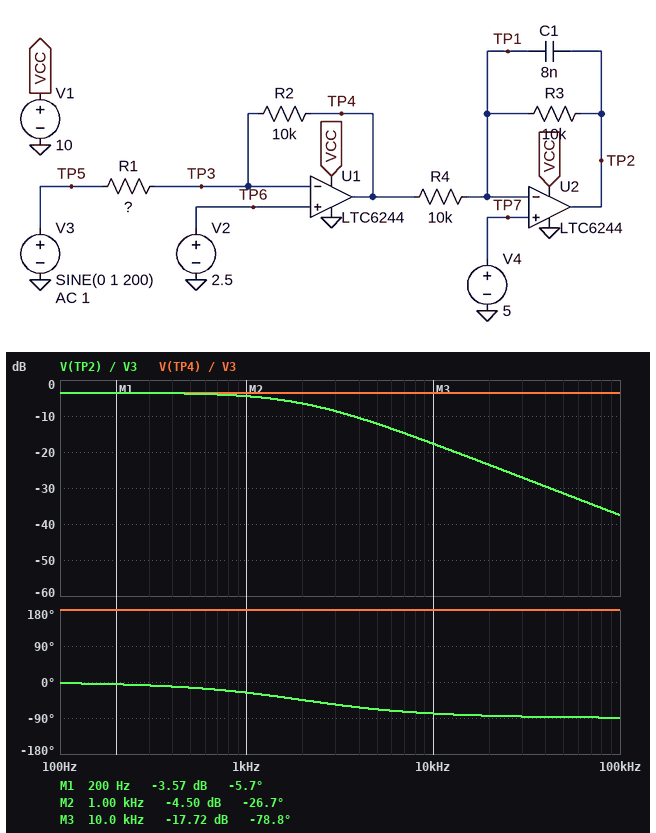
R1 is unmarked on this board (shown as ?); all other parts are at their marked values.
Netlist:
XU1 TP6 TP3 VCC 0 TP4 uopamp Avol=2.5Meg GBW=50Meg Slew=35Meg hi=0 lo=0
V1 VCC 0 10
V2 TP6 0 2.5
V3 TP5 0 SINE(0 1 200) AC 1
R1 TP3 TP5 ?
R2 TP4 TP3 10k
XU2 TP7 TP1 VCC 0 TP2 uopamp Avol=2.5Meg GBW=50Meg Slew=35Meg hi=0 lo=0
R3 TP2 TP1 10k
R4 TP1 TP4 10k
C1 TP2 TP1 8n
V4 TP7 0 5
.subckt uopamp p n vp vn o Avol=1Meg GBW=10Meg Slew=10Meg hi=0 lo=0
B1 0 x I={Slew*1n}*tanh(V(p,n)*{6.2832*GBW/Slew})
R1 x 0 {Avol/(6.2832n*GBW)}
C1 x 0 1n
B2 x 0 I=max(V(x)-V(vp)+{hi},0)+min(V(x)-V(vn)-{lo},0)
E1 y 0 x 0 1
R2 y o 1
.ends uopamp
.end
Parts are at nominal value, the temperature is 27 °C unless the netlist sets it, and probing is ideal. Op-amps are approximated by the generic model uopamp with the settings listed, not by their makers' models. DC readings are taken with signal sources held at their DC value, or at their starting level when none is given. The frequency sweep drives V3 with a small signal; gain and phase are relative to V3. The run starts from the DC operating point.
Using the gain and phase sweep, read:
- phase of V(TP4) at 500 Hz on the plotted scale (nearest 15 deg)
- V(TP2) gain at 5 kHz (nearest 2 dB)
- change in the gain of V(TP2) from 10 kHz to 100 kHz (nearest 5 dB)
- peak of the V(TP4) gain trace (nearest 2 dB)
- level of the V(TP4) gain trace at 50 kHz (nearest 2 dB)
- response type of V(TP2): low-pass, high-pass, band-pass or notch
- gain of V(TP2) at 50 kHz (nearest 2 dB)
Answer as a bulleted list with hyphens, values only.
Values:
- 180 deg
- -12 dB
- -20 dB
- -4 dB
- -4 dB
- low-pass
- -32 dB
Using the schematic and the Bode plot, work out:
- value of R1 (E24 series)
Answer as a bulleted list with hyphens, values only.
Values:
- 15 kΩ
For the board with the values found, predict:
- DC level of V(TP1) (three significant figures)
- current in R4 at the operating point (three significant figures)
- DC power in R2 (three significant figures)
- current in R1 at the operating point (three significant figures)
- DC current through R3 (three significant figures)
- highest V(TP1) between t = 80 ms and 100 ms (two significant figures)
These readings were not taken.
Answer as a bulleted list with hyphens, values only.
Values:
- 5.00 V
- 83.3 µA
- 278 µW
- 167 µA
- 83.3 µA
- 5.0 V
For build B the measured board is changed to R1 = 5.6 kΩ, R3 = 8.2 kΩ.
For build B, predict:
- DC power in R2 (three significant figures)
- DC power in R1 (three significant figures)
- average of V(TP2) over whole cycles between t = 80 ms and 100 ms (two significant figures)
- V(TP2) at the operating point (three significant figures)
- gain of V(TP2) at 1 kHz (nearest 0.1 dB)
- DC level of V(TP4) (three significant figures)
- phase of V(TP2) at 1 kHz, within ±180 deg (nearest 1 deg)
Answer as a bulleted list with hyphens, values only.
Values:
- 1.99 mW
- 1.12 mW
- 3.4 V
- 3.39 V
- 2.6 dB
- 6.96 V
- -22 deg
